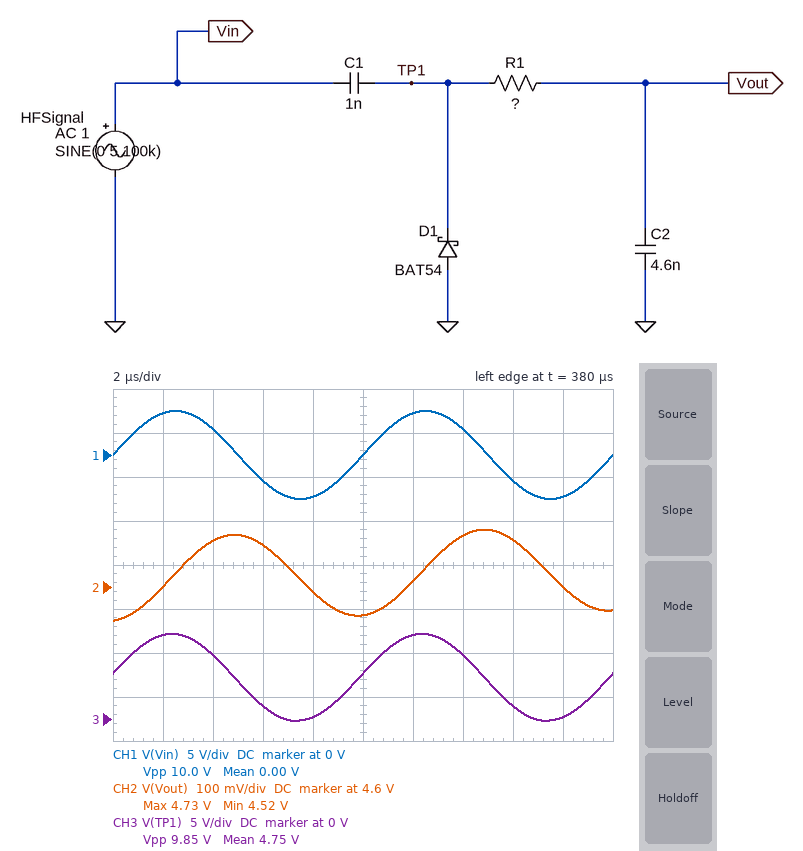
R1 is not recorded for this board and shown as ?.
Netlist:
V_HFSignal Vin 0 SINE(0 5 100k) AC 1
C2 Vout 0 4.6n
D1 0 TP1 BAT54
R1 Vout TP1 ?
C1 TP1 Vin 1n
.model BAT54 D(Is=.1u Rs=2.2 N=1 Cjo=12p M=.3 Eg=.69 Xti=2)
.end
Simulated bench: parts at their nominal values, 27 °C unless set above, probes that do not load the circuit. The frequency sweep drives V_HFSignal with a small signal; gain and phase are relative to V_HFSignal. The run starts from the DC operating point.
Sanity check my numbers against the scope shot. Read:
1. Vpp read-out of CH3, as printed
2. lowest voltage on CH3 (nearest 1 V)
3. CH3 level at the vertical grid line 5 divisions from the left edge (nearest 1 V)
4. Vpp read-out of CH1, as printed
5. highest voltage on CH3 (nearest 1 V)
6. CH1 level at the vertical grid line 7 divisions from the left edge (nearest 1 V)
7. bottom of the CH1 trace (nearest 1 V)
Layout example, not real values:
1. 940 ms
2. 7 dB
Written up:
1. 9.85 V
2. 0 V
3. 5 V
4. 10.0 V
5. 10 V
6. 3 V
7. -5 V
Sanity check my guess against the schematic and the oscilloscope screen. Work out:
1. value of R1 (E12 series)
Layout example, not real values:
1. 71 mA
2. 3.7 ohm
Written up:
1. 18 kΩ
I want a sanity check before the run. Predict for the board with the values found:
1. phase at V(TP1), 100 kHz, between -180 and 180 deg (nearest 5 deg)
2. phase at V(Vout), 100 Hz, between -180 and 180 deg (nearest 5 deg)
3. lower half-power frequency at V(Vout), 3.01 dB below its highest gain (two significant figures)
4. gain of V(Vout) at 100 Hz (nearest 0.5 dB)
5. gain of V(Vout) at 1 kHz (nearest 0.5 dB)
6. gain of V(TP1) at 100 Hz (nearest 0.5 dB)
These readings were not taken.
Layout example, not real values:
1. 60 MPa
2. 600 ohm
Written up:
1. 5 deg
2. 45 deg
3. 100 Hz
4. -18.5 dB
5. -15.5 dB
6. -18.5 dB
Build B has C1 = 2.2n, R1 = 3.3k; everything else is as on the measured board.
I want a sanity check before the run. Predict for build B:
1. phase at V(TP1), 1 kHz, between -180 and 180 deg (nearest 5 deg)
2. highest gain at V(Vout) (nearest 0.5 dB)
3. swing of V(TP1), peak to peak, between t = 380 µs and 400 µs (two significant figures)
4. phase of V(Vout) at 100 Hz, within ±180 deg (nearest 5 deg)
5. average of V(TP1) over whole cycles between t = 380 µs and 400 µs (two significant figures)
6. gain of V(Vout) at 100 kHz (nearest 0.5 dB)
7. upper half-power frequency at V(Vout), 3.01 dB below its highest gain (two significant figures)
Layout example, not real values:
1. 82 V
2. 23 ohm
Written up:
1. 10 deg
2. -10.0 dB
3. 9.5 V
4. 40 deg
5. 4.6 V
6. -20.0 dB
7. 33 kHz
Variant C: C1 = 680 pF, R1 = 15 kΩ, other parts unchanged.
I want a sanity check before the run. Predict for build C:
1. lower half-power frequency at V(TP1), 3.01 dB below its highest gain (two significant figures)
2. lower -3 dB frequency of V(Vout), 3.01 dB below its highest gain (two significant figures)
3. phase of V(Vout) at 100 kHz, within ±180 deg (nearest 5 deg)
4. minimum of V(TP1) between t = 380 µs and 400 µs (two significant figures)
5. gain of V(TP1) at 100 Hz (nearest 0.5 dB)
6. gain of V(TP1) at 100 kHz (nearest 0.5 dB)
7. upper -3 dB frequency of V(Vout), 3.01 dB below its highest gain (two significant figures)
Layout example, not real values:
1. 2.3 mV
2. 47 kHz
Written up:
1. 18 kHz
2. 110 Hz
3. -80 deg
4. -190 mV
5. -21.5 dB
6. -0.5 dB
7. 19 kHz
